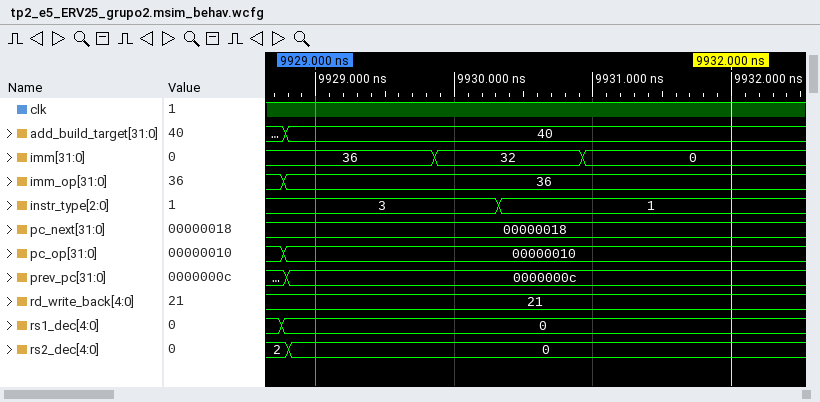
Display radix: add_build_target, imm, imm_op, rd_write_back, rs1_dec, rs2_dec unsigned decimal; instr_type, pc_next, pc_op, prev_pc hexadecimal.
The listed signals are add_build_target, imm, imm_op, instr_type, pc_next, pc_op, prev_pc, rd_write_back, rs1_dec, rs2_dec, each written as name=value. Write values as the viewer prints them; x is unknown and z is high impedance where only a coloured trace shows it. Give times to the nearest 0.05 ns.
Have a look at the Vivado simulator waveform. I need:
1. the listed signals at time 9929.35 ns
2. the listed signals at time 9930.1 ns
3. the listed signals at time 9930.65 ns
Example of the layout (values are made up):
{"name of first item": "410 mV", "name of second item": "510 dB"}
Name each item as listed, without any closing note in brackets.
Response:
{"the listed signals at time 9929.35 ns": "add_build_target=40, imm=36, imm_op=36, instr_type=3, pc_next=00000018, pc_op=00000010, prev_pc=0000000c, rd_write_back=21, rs1_dec=0, rs2_dec=0", "the listed signals at time 9930.1 ns": "add_build_target=40, imm=32, imm_op=36, instr_type=3, pc_next=00000018, pc_op=00000010, prev_pc=0000000c, rd_write_back=21, rs1_dec=0, rs2_dec=0", "the listed signals at time 9930.65 ns": "add_build_target=40, imm=32, imm_op=36, instr_type=1, pc_next=00000018, pc_op=00000010, prev_pc=0000000c, rd_write_back=21, rs1_dec=0, rs2_dec=0"}
